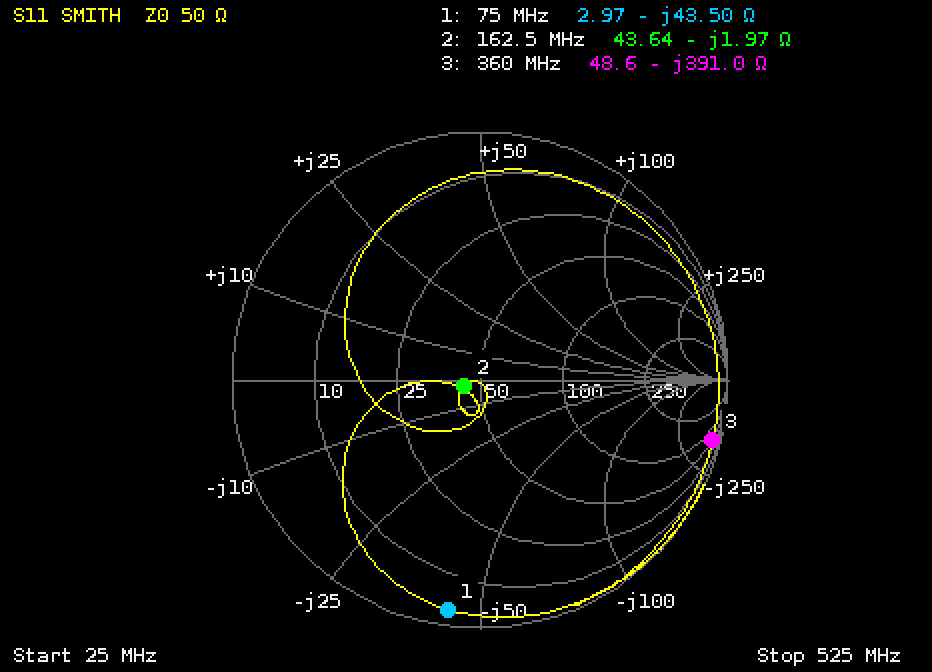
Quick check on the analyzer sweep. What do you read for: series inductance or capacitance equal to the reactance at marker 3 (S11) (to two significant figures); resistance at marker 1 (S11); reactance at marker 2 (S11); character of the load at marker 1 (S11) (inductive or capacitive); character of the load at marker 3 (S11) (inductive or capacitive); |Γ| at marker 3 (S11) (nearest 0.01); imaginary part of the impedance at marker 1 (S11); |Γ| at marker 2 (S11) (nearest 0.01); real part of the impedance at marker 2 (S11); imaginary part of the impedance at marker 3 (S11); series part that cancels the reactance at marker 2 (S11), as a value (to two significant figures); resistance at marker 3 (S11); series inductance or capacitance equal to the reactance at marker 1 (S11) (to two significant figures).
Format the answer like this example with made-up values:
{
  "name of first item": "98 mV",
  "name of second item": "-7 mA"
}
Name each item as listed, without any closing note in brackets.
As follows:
{
  "series inductance or capacitance equal to the reactance at marker 3 (S11)": "1.1 pF",
  "resistance at marker 1": "2.97 Ω",
  "reactance at marker 2": "-1.97 Ω",
  "character of the load at marker 1 (S11)": "capacitive",
  "character of the load at marker 3 (S11)": "capacitive",
  "|Γ| at marker 3 (S11)": "0.97",
  "imaginary part of the impedance at marker 1": "-43.50 Ω",
  "|Γ| at marker 2 (S11)": "0.07",
  "real part of the impedance at marker 2": "43.64 Ω",
  "imaginary part of the impedance at marker 3": "-391.0 Ω",
  "series part that cancels the reactance at marker 2 (S11), as a value": "1.9 nH",
  "resistance at marker 3": "48.6 Ω",
  "series inductance or capacitance equal to the reactance at marker 1 (S11)": "49 pF"
}
